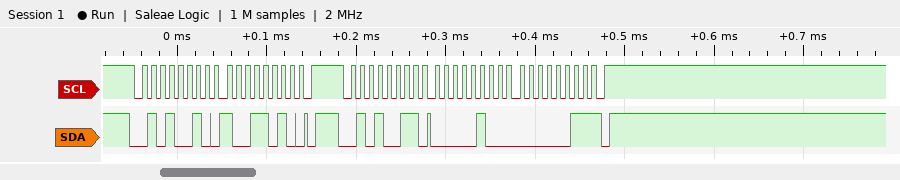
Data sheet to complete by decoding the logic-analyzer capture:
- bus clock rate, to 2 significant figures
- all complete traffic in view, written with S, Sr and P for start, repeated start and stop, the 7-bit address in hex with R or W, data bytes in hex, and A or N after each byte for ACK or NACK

100 kHz
S 29W A 9A A P S 29R A 04 A 03 N P
